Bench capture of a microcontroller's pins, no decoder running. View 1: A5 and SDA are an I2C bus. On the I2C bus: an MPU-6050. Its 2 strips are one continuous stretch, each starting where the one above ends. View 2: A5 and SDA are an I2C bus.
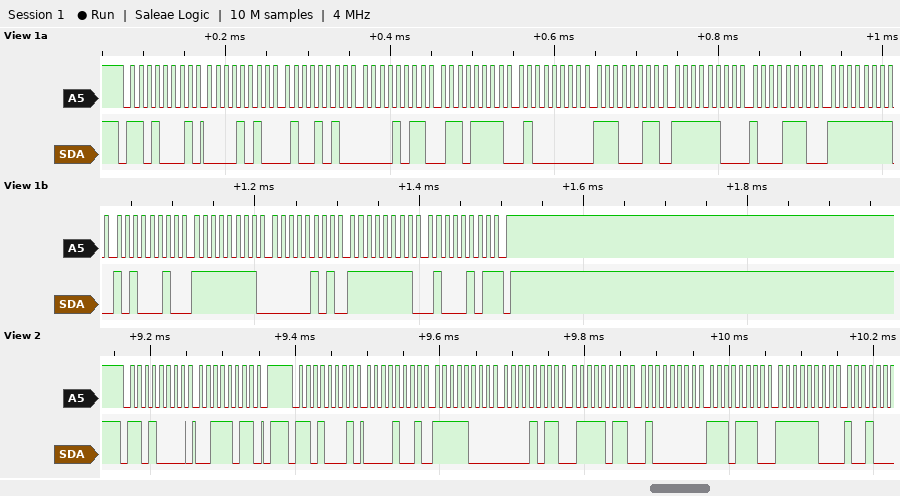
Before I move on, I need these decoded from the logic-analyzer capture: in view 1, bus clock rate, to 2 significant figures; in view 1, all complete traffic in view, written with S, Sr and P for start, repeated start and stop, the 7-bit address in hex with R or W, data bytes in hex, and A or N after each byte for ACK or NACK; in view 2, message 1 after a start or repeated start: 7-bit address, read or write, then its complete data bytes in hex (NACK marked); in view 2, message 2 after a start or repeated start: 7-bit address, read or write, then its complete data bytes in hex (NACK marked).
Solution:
100 kHz
S 68R A 0A A 4A A 0B A 6F A 40 A E3 A FC A 8E A FF A A2 A FF A 05 A FF A 45 N P
0x68 write: 3B
0x68 read: 09 F8 0B 7B 40 EE FC
